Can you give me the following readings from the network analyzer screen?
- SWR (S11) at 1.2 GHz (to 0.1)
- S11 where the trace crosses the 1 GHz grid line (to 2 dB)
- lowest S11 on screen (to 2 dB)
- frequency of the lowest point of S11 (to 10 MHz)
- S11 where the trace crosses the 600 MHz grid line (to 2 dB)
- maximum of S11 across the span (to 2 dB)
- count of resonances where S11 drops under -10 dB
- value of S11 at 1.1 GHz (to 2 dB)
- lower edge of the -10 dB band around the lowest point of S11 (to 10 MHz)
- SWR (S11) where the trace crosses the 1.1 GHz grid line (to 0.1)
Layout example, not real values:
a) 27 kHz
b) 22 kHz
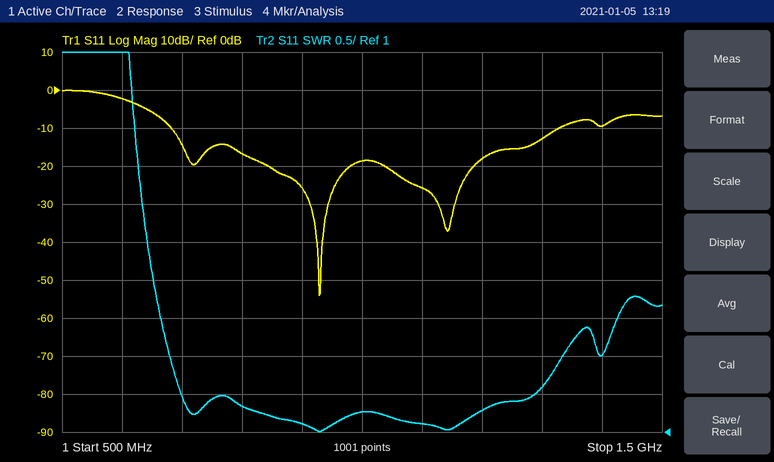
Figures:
a) 1.3
b) -18 dB
c) -54 dB
d) 930 MHz
e) -2 dB
f) 0 dB
g) 3
h) -26 dB
i) 680 MHz
j) 1.1
